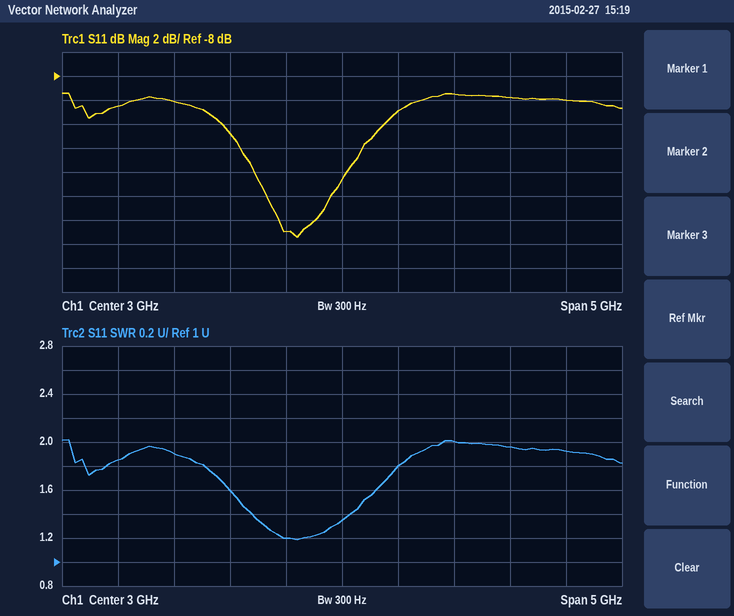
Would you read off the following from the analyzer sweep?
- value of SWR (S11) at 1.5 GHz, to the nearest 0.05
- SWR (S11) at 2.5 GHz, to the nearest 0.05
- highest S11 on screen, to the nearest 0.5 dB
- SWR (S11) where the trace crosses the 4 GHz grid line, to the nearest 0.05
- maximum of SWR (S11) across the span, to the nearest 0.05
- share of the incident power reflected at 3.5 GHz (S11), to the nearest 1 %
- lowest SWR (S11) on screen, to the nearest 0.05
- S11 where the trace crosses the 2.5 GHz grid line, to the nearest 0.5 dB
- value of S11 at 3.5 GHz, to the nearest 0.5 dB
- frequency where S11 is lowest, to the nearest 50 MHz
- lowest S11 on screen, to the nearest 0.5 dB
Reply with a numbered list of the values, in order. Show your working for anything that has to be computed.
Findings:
1. 1.90
2. 1.20
3. -9.5 dB
4. 2.00
5. 2.00
6. 10^(-11/10) ≈ 8 %
7. 1.20
8. -21.0 dB
9. -11.0 dB
10. 2.60 GHz
11. -21.5 dB
